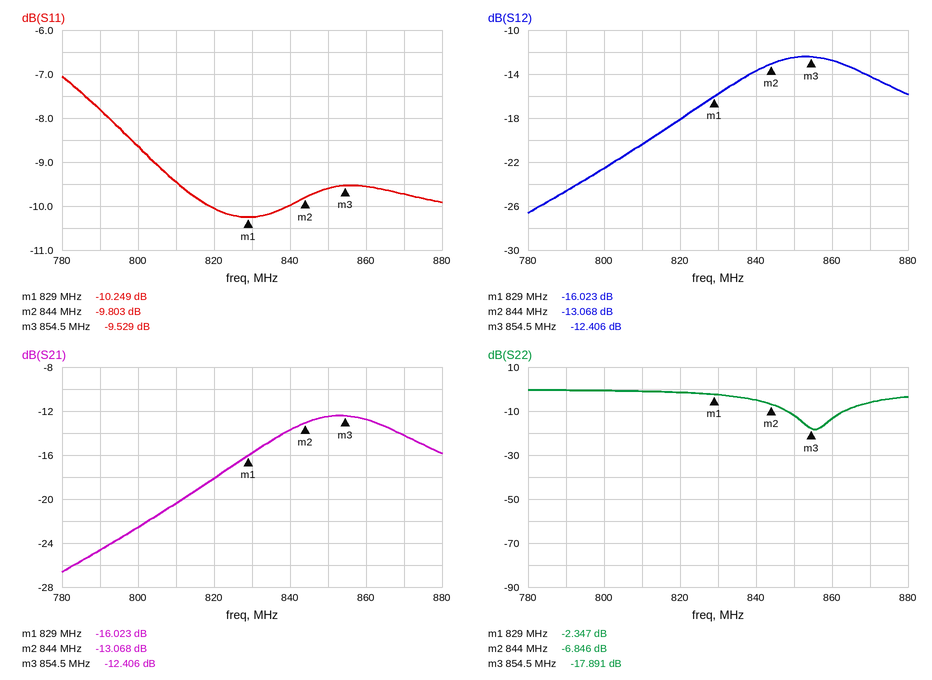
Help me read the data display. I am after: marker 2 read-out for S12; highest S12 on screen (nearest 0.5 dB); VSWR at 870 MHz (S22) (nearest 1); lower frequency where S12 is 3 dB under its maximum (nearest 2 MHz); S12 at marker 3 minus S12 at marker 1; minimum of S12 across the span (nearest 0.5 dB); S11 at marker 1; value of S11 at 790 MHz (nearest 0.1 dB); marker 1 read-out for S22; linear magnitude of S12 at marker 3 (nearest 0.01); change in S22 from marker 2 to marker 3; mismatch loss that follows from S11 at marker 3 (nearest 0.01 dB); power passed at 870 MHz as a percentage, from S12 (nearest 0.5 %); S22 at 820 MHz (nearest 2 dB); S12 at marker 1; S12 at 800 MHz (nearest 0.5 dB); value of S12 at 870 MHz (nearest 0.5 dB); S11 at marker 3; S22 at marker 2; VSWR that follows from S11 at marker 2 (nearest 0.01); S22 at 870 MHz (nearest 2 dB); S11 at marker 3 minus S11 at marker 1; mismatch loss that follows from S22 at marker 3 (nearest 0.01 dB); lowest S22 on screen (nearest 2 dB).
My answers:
-13.068 dB
-12.5 dB
3
832 MHz
3.617 dB
-26.5 dB
-10.249 dB
-7.8 dB
-2.347 dB
0.24
-11.045 dB
0.51 dB
4.0 %
-2 dB
-16.023 dB
-22.5 dB
-14.0 dB
-9.529 dB
-6.846 dB
1.96
-6 dB
0.720 dB
0.07 dB
-18 dB
